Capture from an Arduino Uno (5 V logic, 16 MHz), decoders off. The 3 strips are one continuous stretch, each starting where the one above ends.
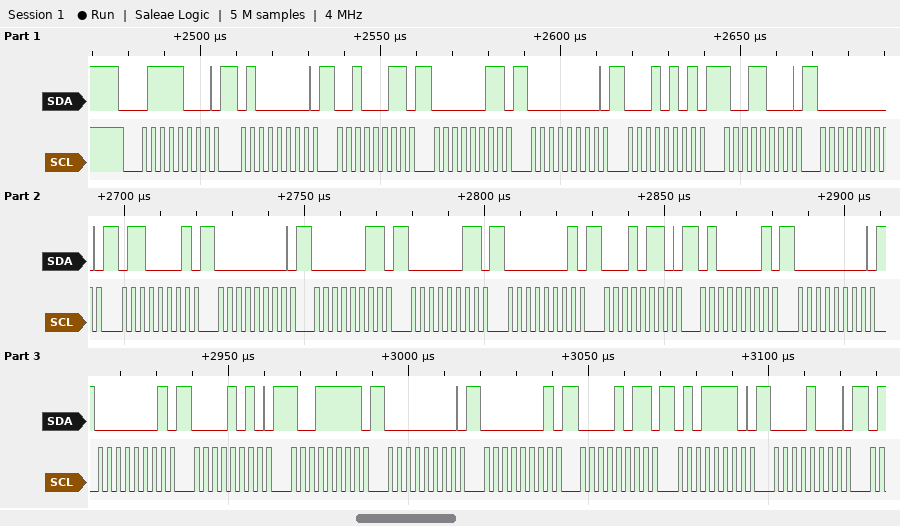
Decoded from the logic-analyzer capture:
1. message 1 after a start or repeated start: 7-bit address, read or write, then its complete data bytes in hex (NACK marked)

0x3C write: 40 23 03 00 15 98 00 61 00 03 03 01 16 41 00 01 0A 9F 00 01 0B 5E 08
